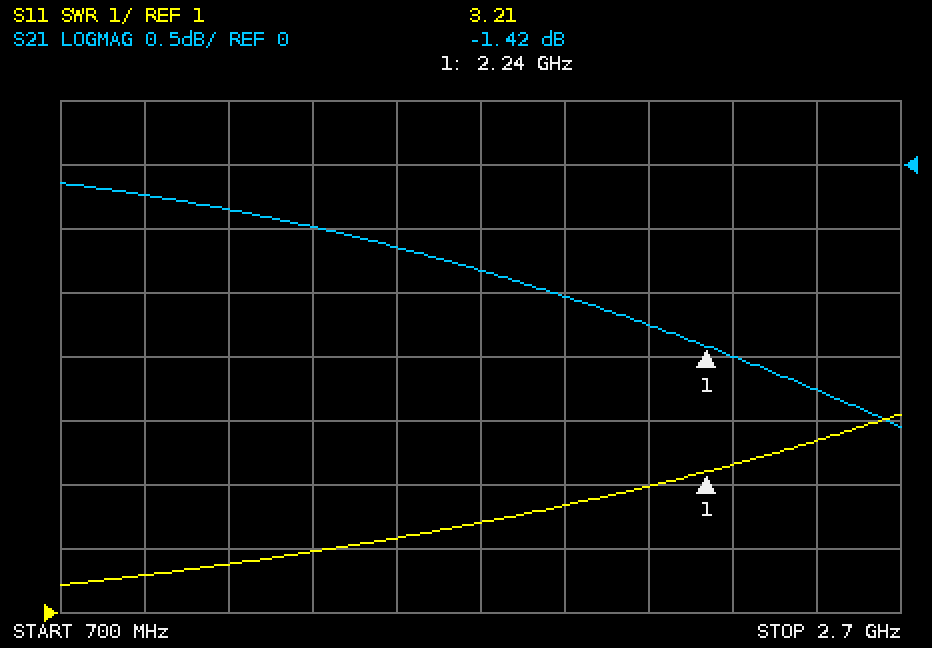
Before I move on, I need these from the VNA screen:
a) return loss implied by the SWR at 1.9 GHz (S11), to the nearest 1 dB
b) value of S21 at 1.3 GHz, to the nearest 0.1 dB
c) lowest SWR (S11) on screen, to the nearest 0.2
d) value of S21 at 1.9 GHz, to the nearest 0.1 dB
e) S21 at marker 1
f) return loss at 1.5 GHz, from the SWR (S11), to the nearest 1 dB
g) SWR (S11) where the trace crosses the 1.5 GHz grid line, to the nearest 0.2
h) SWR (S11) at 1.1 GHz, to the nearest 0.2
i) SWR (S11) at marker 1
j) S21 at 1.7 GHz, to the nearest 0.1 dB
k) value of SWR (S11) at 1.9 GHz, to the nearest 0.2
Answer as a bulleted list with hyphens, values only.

- 7 dB
- -0.5 dB
- 1.4
- -1.0 dB
- -1.42 dB
- 9 dB
- 2.2
- 1.8
- 3.21
- -0.8 dB
- 2.6
